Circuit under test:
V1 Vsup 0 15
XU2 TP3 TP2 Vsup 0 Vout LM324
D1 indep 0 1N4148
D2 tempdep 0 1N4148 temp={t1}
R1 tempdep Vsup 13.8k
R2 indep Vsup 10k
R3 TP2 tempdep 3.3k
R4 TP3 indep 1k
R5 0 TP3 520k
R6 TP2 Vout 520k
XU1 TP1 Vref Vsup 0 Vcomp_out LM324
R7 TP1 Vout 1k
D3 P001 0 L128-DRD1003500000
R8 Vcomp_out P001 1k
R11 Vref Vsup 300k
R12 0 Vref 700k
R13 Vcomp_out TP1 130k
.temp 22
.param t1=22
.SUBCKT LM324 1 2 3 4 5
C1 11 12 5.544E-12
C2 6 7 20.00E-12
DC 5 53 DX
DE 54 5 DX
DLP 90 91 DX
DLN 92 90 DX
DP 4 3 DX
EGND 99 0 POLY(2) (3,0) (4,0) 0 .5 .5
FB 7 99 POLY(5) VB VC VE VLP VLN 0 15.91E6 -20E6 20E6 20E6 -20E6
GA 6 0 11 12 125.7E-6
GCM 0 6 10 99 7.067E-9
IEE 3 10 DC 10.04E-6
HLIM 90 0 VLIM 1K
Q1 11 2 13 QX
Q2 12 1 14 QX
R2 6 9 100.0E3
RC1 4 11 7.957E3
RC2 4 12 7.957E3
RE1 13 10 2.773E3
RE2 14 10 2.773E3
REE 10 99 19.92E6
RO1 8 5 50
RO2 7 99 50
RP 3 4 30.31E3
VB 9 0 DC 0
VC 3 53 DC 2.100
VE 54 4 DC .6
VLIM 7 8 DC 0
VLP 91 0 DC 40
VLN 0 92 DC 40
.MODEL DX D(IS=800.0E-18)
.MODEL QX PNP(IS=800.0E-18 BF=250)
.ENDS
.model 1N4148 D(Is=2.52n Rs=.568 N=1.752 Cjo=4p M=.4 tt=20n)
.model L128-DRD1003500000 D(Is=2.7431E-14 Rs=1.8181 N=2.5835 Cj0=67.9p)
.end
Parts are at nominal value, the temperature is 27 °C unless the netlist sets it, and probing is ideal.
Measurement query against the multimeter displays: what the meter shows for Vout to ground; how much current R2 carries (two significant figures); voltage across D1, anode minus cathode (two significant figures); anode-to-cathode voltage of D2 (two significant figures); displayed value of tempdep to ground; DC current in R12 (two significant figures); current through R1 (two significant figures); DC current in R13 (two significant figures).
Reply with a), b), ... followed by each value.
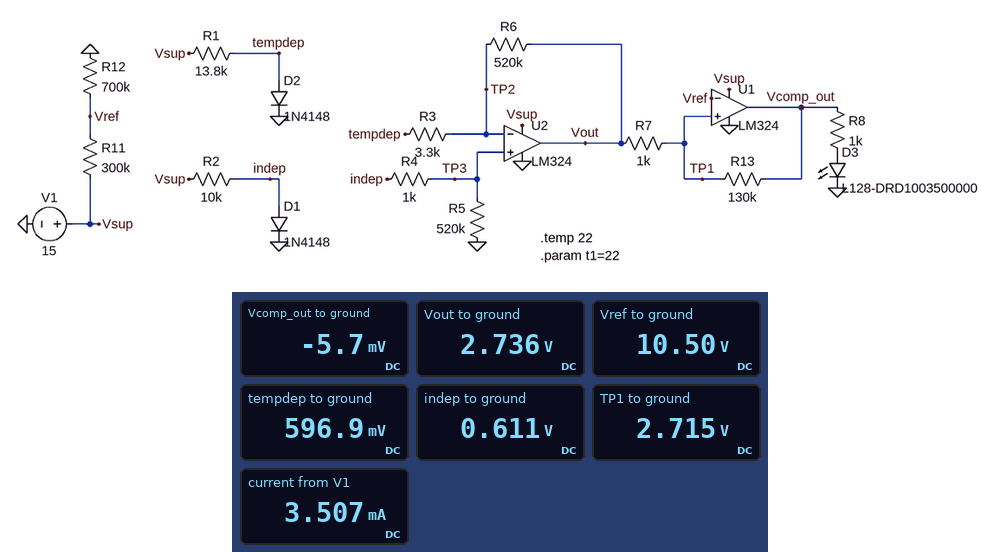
a) 2.736 V
b) 1.4 mA
c) 610 mV
d) 600 mV
e) 596.9 mV
f) 15 µA
g) 1.0 mA
h) 21 µA
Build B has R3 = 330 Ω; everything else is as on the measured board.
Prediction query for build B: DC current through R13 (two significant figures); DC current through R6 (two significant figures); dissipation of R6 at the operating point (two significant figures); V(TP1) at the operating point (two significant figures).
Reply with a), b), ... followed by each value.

a) 550 nA
b) 25 µA
c) 320 µW
d) 13 V
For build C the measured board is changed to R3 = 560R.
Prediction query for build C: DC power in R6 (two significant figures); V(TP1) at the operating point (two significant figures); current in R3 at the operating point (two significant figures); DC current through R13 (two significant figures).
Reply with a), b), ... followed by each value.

a) 270 µW
b) 12 V
c) 23 µA
d) 8.7 µA
